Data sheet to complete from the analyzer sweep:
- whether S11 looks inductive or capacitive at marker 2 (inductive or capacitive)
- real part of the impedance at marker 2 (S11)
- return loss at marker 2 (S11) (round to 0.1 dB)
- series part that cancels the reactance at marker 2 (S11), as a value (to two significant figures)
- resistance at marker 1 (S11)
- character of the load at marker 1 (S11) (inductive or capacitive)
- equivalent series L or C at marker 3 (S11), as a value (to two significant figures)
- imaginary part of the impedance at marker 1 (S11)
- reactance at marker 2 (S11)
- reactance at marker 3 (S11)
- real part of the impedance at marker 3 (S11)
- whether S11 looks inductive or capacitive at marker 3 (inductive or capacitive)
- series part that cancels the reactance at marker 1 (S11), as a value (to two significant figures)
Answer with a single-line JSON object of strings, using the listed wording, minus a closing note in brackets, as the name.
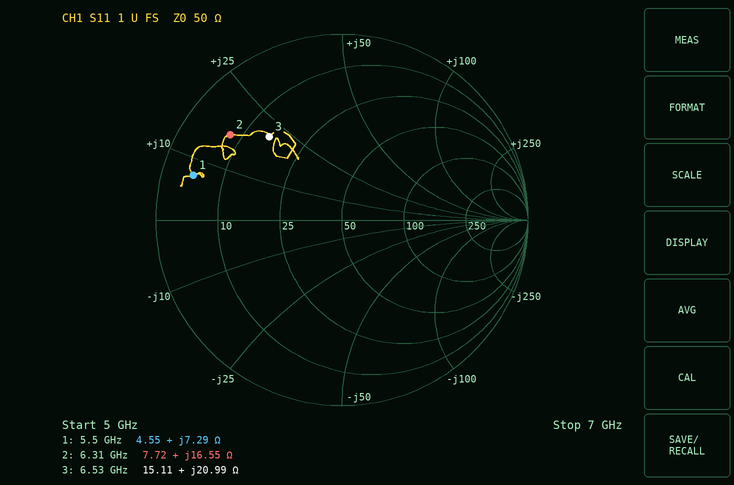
{"whether S11 looks inductive or capacitive at marker 2": "inductive", "real part of the impedance at marker 2": "7.72 Ω", "return loss at marker 2 (S11)": "2.4 dB", "series part that cancels the reactance at marker 2 (S11), as a value": "1.5 pF", "resistance at marker 1": "4.55 Ω", "character of the load at marker 1 (S11)": "inductive", "equivalent series L or C at marker 3 (S11), as a value": "510 pH", "imaginary part of the impedance at marker 1": "+7.29 Ω", "reactance at marker 2": "+16.55 Ω", "reactance at marker 3": "+20.99 Ω", "real part of the impedance at marker 3": "15.11 Ω", "whether S11 looks inductive or capacitive at marker 3": "inductive", "series part that cancels the reactance at marker 1 (S11), as a value": "4.0 pF"}
